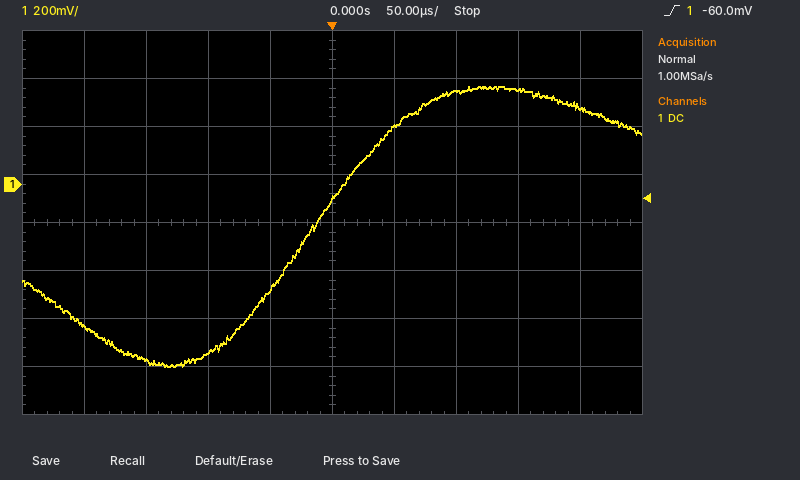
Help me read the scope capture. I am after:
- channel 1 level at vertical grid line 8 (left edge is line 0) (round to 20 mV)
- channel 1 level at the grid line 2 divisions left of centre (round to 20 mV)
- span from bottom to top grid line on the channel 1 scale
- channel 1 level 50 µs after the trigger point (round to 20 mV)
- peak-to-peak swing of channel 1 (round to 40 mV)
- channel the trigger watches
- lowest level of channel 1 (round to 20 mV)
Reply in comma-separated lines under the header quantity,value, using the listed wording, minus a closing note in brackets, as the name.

quantity,value
channel 1 level at vertical grid line 8 (left edge is line 0),400 mV
channel 1 level at the grid line 2 divisions left of centre,-700 mV
span from bottom to top grid line on the channel 1 scale,1.6 V
channel 1 level 50 µs after the trigger point,240 mV
peak-to-peak swing of channel 1,1.16 V
channel the trigger watches,channel 1
lowest level of channel 1,-760 mV
